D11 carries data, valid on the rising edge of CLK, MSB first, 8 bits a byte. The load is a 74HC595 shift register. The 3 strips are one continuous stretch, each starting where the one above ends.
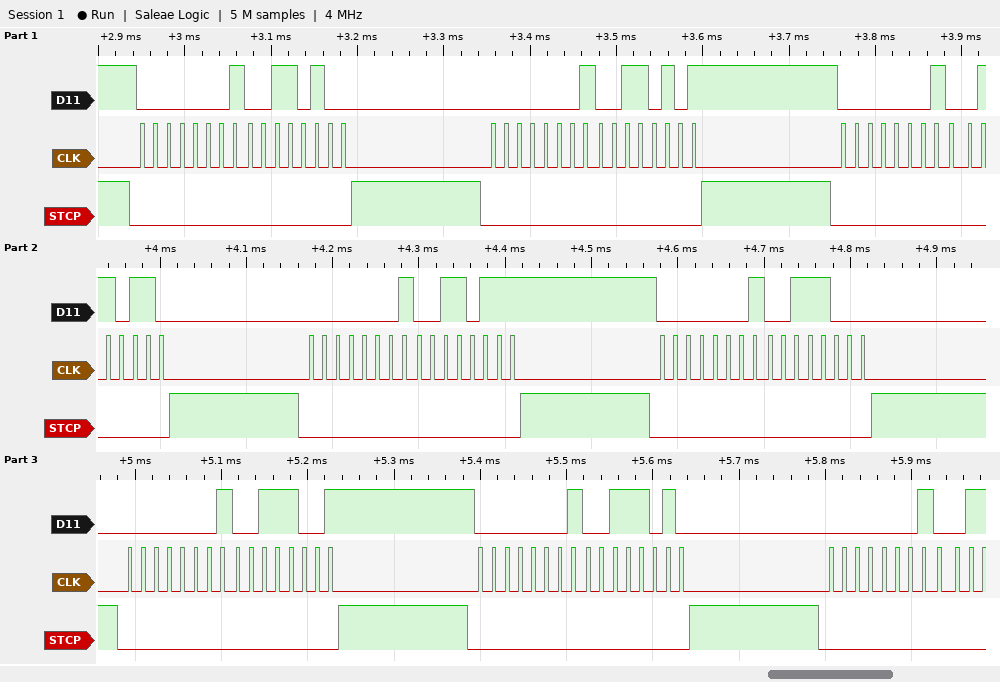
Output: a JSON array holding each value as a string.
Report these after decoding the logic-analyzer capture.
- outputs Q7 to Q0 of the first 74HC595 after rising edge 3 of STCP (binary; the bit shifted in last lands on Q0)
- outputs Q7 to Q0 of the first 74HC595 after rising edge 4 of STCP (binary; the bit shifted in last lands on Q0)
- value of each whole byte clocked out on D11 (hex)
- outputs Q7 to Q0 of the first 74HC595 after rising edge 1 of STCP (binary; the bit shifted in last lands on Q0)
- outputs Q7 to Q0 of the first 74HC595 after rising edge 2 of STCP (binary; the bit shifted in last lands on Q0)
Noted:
["00110110", "00110111", "0x01 0x34 0x01 0x35 0x01 0x36 0x01 0x37 0x01 0x38 0x01 0x39 0x01 0x3A 0x01", "00110100", "00110101"]
